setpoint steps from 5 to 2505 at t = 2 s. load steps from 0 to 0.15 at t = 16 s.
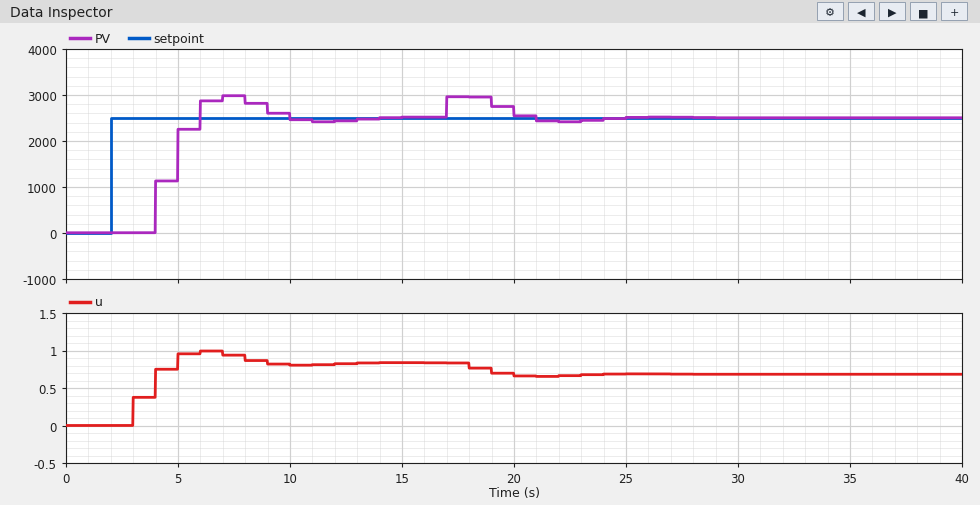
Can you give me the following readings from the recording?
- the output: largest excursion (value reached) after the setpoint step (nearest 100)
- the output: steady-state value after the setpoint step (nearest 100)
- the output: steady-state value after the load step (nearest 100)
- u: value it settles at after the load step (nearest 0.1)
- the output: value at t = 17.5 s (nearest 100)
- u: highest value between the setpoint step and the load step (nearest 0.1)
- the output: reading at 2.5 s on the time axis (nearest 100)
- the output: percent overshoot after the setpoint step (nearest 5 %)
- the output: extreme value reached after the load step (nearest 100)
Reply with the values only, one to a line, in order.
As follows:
3000
2500
2500
0.7
3000
1.0
0
20 %
3000
